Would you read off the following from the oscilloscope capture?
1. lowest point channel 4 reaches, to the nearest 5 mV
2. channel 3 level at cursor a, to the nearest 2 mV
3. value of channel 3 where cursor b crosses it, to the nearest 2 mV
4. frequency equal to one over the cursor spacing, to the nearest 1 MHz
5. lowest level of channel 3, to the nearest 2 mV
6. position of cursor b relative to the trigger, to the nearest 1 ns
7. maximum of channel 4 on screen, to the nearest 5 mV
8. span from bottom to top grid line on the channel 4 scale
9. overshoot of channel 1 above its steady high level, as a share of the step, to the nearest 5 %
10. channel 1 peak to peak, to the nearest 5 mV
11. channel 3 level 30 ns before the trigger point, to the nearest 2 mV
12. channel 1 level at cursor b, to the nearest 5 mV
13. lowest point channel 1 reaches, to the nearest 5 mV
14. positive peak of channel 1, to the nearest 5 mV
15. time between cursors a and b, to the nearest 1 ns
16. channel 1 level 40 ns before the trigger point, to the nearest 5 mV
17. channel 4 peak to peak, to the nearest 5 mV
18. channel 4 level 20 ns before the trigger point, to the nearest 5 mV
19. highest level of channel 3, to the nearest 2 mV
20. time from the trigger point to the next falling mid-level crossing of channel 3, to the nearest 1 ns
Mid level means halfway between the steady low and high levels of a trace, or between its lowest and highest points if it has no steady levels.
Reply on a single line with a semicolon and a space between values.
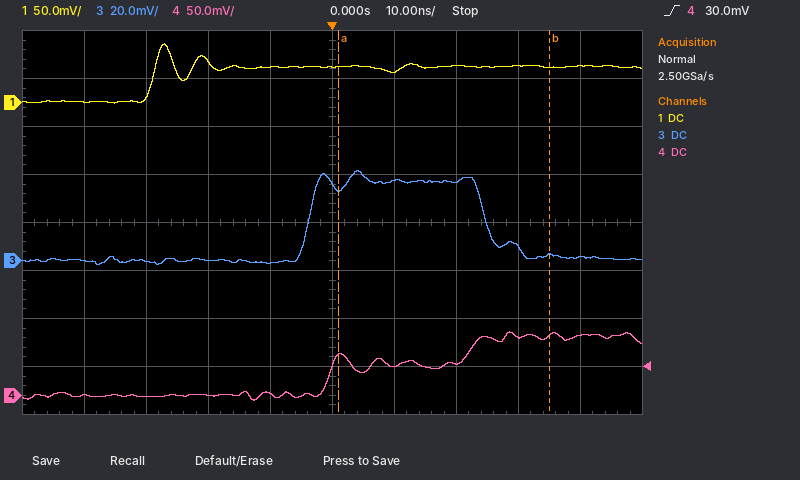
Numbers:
-5 mV; 30 mV; 2 mV; 29 MHz; -2 mV; +35 ns; 65 mV; 400 mV; 65 %; 60 mV; 0 mV; 35 mV; 0 mV; 60 mV; 34 ns; 0 mV; 70 mV; 0 mV; 38 mV; 25 ns
